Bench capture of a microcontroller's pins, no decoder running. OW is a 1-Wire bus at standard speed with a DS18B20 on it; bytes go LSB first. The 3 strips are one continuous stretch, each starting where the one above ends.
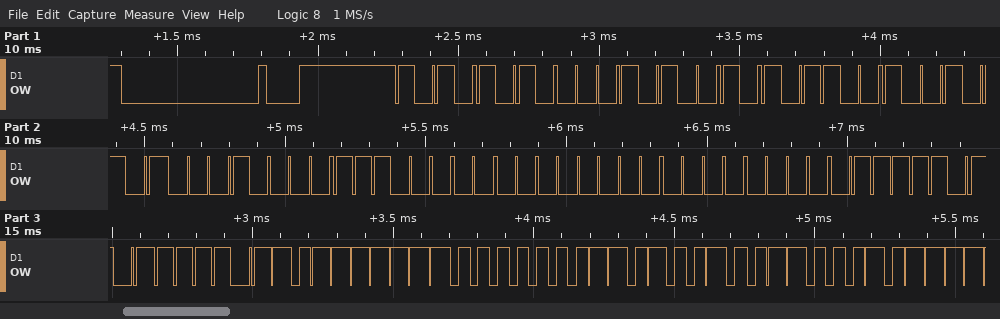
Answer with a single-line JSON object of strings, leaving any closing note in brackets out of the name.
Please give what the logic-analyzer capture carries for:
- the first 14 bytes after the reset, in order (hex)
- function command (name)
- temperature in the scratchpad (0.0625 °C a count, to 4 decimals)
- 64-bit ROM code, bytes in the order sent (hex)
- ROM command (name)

{"the first 14 bytes after the reset, in order": "55 28 35 A9 08 07 00 00 BE BE FD 01 4B 46", "function command": "Read Scratchpad", "temperature in the scratchpad": "31.8125 °C", "64-bit ROM code, bytes in the order sent": "28 35 A9 08 07 00 00 BE", "ROM command": "Match ROM"}
